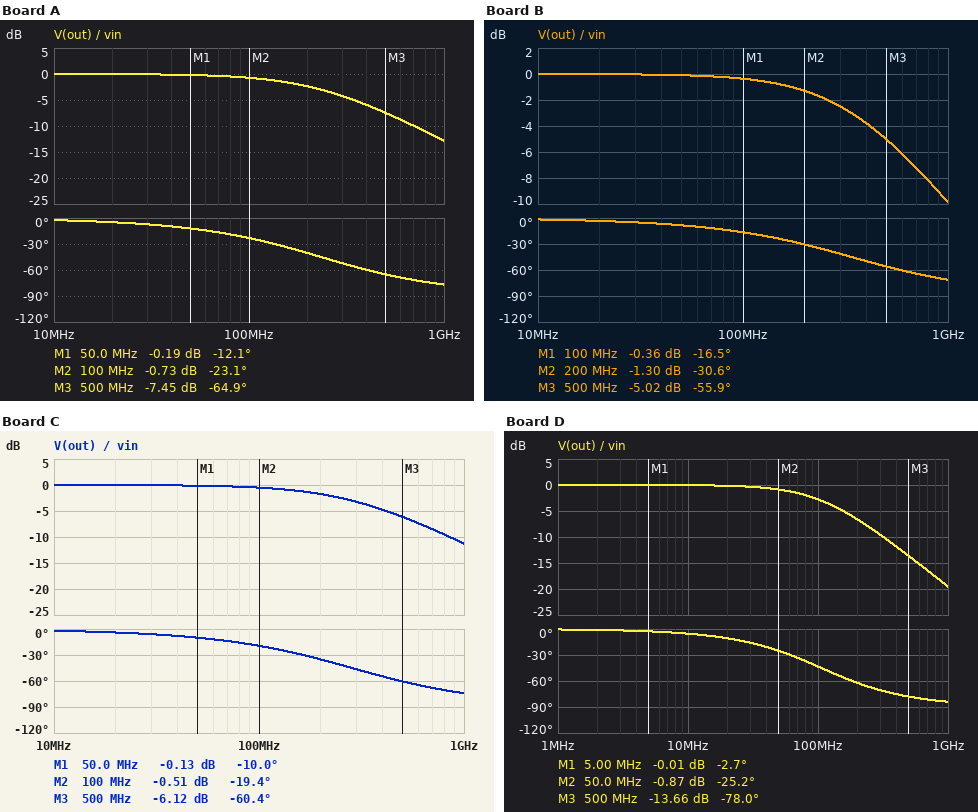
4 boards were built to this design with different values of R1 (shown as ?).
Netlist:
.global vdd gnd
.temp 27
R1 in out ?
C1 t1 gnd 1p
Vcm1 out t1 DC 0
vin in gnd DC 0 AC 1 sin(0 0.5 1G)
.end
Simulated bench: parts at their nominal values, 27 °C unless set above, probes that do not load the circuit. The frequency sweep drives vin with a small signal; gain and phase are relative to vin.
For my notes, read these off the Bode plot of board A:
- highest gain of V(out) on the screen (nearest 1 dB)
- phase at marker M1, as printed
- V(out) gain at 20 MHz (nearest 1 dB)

0 dB
-12.1 deg
0 dB
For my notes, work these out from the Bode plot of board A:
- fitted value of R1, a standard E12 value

680 Ω
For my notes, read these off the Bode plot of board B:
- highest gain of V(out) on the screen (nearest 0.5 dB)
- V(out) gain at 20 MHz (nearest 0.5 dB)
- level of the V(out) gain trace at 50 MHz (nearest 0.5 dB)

0 dB
0 dB
0 dB
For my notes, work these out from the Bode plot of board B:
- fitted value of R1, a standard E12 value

470 Ω
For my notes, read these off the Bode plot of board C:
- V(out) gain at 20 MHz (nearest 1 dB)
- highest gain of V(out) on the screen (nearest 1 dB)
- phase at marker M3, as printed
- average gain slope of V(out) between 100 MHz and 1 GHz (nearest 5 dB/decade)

0 dB
0 dB
-60.4 deg
-10 dB/decade
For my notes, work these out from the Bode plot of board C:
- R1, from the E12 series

560 Ω
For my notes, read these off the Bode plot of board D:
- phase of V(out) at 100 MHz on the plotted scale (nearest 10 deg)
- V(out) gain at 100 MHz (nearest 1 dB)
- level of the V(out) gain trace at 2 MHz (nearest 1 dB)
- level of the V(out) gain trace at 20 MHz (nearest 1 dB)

-40 deg
-3 dB
0 dB
0 dB
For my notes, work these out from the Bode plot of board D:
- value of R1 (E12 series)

1.5 kΩ
